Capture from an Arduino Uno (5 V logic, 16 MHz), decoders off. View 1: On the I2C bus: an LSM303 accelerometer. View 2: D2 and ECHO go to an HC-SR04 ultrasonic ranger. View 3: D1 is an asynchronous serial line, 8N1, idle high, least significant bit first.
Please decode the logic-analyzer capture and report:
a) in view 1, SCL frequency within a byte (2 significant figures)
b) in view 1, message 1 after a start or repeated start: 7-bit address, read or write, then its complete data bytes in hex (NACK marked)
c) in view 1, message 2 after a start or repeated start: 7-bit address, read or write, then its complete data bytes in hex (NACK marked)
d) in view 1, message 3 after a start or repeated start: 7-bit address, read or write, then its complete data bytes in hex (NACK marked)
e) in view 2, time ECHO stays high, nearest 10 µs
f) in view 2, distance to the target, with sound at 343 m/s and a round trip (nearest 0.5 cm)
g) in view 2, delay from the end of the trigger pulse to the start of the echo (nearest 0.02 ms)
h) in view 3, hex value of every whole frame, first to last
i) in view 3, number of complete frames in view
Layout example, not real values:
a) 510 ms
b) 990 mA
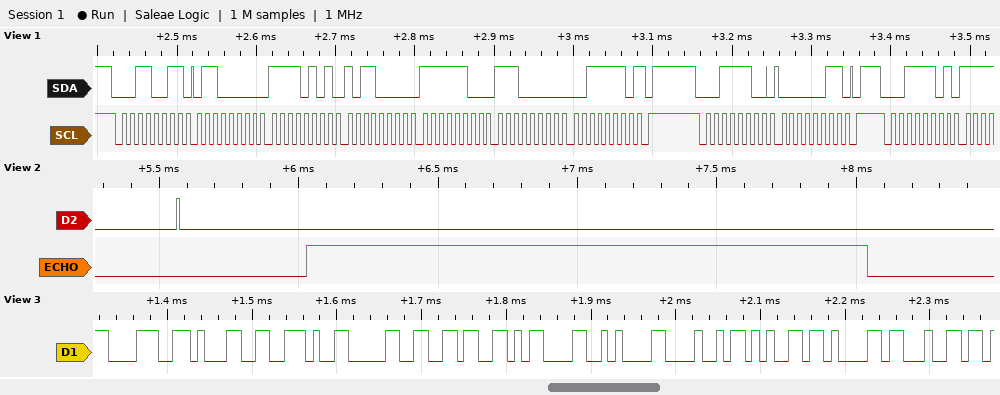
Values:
a) 100 kHz
b) 0x19 read: 60 F5 B0 FC E0 3E NACK
c) 0x1E write: 03
d) 0x1E read
e) 2010 µs
f) 34.5 cm
g) 0.46 ms
h) 38 31 2E 30 36 0D 0A 48 65 61 64
i) 11
